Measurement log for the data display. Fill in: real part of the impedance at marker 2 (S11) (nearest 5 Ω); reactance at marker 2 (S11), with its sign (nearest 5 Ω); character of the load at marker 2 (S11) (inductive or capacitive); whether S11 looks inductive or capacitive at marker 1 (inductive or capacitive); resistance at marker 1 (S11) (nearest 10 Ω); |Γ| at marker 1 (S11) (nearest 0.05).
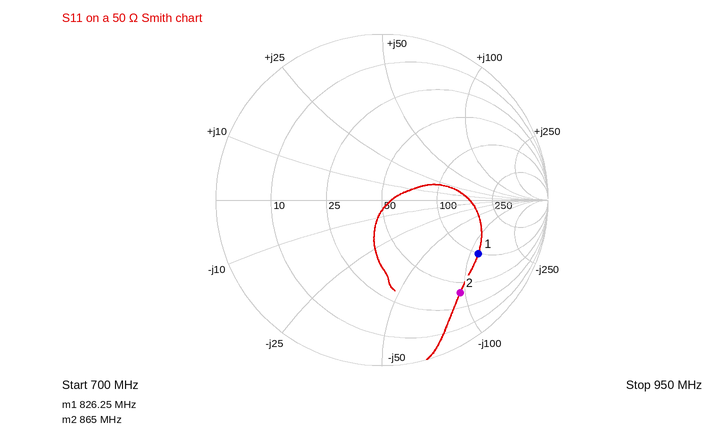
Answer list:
40 Ω
-95 Ω
capacitive
capacitive
100 Ω
0.65
